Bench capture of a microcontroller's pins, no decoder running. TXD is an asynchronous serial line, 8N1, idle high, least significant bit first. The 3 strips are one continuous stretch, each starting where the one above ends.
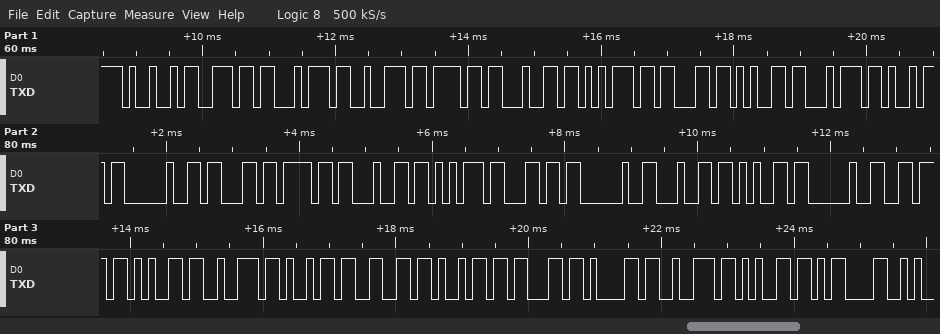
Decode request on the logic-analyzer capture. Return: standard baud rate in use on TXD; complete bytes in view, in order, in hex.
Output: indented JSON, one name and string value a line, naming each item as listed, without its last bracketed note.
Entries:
{
  "standard baud rate in use on TXD": "9600 baud",
  "complete bytes in view, in order, in hex": "49 6E 74 72 6F 64 75 63 65 74 69 20 63 6F 64 75 6C 20 64 65 20 76 65 72 69 66 69 63 61 72 65 0D"
}
